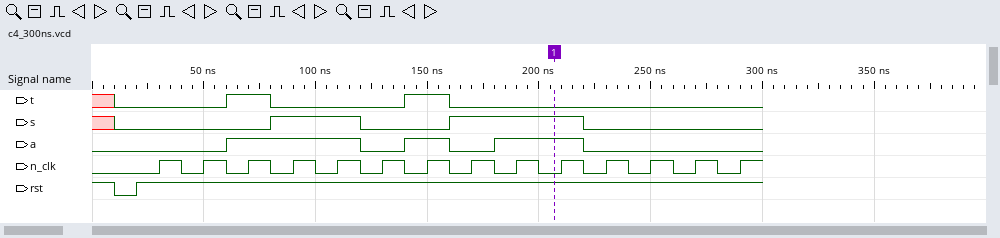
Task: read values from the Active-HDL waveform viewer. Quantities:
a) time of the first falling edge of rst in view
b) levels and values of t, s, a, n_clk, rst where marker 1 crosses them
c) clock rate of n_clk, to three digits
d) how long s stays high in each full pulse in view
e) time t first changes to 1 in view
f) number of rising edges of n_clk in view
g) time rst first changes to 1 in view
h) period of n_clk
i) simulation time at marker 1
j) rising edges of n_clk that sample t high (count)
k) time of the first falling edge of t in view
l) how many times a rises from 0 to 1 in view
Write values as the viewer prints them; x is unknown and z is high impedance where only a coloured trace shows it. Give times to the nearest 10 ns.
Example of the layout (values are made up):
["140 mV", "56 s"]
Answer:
["10 ns", "t=0, s=1, a=1, n_clk=0, rst=1", "50.0 MHz", "40 ns, 60 ns", "60 ns", "14", "20 ns", "20 ns", "210 ns", "2", "80 ns", "3"]
